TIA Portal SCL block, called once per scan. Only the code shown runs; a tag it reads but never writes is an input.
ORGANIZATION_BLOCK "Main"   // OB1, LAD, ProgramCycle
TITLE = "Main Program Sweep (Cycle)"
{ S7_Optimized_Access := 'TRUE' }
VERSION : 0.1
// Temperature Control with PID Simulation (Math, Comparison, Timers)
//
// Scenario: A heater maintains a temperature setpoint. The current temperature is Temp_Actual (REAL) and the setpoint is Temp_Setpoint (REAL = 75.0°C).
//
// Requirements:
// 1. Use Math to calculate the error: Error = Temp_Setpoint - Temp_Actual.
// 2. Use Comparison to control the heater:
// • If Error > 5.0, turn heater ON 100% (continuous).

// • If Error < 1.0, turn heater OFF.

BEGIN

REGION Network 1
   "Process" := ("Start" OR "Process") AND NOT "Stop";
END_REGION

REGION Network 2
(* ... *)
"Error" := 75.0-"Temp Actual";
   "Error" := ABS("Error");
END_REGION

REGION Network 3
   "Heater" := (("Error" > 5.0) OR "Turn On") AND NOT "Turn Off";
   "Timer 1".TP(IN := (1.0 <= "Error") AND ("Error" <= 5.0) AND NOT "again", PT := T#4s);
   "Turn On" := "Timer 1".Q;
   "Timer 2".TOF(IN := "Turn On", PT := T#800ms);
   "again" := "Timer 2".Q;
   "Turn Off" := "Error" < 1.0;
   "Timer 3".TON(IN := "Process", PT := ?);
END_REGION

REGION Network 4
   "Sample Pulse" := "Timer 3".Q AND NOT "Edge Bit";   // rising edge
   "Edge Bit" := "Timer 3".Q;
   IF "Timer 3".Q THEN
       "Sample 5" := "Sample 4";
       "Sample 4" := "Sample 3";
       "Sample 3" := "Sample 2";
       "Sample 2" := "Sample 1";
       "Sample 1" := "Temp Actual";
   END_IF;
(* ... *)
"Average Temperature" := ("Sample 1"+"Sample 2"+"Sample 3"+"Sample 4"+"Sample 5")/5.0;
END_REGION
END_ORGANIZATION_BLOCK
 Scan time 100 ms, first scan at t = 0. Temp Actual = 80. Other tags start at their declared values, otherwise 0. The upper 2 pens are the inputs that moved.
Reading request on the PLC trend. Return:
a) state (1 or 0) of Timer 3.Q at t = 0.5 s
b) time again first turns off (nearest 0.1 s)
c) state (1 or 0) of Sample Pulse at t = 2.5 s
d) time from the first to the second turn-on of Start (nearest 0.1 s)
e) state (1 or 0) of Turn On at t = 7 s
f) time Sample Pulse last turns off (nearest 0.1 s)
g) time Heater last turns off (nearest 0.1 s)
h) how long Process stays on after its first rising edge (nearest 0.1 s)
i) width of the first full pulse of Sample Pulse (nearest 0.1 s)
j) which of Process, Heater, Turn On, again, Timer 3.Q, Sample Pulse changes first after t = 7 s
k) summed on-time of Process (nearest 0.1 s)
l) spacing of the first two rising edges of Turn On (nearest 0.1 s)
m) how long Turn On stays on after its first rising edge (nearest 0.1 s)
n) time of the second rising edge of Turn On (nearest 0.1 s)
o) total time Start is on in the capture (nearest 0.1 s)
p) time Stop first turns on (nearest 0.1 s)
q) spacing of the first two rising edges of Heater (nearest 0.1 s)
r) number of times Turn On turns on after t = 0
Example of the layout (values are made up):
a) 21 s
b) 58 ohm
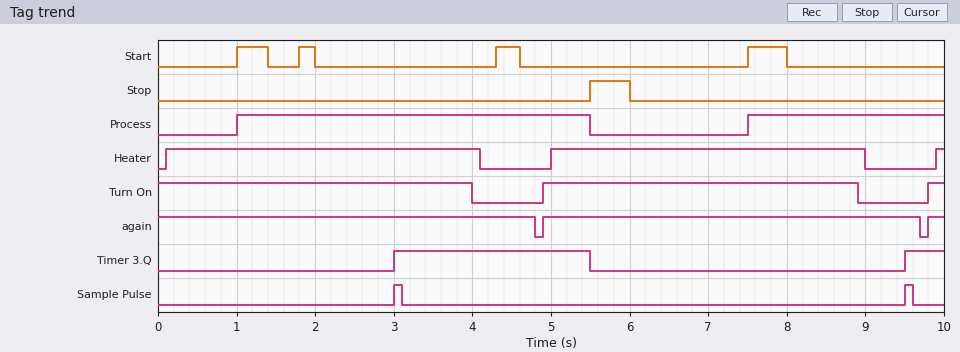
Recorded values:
a) 0
b) 4.8 s
c) 0
d) 0.8 s
e) 1
f) 9.6 s
g) 9.0 s
h) 4.5 s
i) 0.1 s
j) Process
k) 7.0 s
l) 4.9 s
m) 4.0 s
n) 9.8 s
o) 1.4 s
p) 5.5 s
q) 4.9 s
r) 2
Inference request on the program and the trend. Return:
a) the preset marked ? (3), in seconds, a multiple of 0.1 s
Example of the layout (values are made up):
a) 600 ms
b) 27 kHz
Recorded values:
a) 2.0 s
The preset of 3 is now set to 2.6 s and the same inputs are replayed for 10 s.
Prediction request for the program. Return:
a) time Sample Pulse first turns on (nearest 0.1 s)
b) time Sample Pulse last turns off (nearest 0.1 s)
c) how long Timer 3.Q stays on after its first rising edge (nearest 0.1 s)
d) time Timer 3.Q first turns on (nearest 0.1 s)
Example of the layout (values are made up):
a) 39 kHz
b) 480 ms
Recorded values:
a) 3.6 s
b) 3.7 s
c) 1.9 s
d) 3.6 s
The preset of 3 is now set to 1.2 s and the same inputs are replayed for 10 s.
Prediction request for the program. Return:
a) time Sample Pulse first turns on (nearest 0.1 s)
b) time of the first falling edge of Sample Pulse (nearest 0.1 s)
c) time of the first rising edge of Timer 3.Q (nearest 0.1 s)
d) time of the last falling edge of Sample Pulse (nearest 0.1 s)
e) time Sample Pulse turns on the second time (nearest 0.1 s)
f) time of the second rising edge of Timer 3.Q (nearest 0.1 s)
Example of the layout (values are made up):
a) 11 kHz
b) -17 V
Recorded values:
a) 2.2 s
b) 2.3 s
c) 2.2 s
d) 8.8 s
e) 8.7 s
f) 8.7 s
